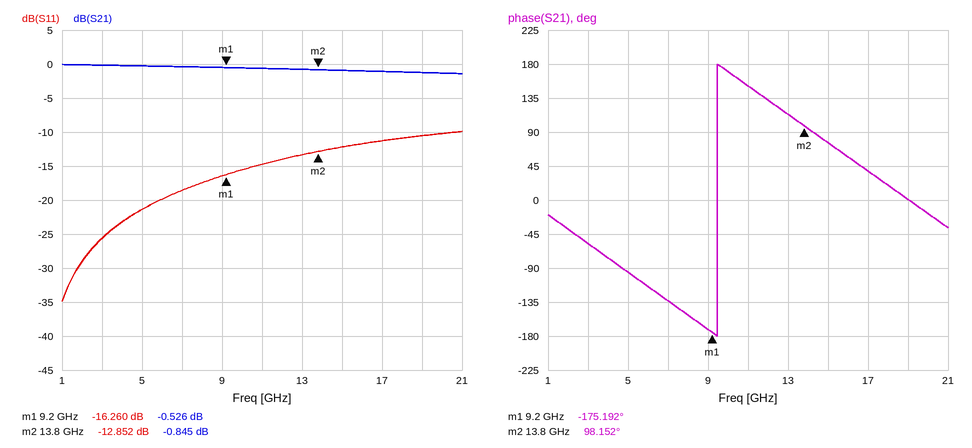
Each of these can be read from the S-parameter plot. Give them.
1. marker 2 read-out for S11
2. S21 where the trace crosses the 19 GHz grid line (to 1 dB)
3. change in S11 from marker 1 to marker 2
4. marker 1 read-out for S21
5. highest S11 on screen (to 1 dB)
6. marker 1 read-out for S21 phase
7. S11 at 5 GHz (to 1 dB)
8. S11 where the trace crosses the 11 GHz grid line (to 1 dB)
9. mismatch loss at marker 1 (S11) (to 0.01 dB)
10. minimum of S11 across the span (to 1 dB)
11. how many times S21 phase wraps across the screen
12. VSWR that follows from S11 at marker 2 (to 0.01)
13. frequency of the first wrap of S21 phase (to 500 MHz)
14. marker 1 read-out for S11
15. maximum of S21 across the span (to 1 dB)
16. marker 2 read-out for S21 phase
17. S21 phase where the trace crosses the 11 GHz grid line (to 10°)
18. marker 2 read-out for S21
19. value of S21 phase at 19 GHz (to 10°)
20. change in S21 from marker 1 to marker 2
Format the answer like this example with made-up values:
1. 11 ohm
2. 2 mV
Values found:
1. -12.852 dB
2. -1 dB
3. 3.408 dB
4. -0.526 dB
5. -10 dB
6. -175.192°
7. -21 dB
8. -15 dB
9. 0.10 dB
10. -35 dB
11. 1
12. 1.59
13. 9.5 GHz
14. -16.260 dB
15. 0 dB
16. 98.152°
17. 150°
18. -0.845 dB
19. 0°
20. -0.319 dB
